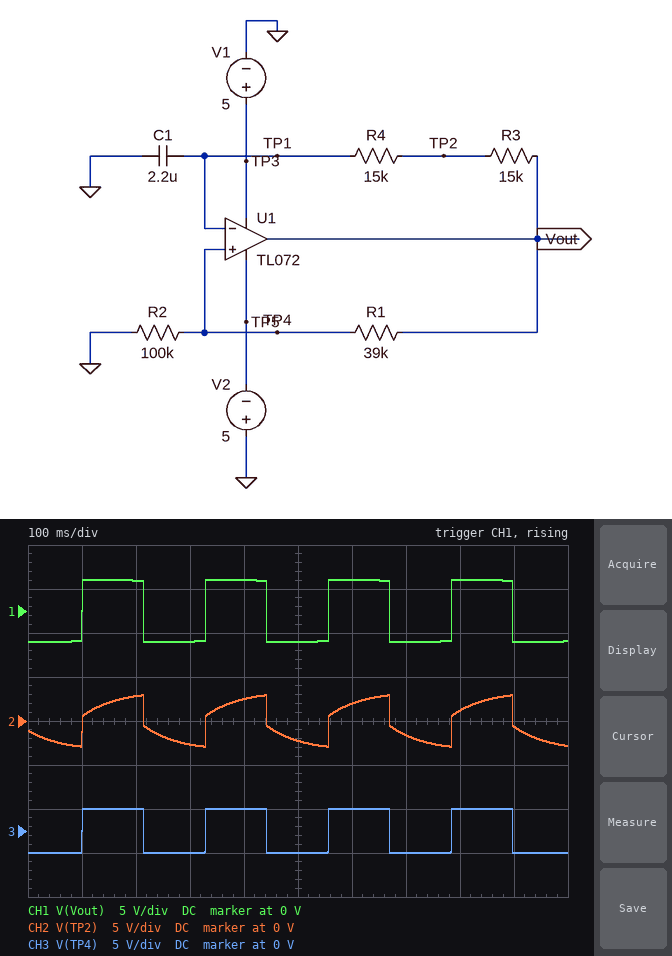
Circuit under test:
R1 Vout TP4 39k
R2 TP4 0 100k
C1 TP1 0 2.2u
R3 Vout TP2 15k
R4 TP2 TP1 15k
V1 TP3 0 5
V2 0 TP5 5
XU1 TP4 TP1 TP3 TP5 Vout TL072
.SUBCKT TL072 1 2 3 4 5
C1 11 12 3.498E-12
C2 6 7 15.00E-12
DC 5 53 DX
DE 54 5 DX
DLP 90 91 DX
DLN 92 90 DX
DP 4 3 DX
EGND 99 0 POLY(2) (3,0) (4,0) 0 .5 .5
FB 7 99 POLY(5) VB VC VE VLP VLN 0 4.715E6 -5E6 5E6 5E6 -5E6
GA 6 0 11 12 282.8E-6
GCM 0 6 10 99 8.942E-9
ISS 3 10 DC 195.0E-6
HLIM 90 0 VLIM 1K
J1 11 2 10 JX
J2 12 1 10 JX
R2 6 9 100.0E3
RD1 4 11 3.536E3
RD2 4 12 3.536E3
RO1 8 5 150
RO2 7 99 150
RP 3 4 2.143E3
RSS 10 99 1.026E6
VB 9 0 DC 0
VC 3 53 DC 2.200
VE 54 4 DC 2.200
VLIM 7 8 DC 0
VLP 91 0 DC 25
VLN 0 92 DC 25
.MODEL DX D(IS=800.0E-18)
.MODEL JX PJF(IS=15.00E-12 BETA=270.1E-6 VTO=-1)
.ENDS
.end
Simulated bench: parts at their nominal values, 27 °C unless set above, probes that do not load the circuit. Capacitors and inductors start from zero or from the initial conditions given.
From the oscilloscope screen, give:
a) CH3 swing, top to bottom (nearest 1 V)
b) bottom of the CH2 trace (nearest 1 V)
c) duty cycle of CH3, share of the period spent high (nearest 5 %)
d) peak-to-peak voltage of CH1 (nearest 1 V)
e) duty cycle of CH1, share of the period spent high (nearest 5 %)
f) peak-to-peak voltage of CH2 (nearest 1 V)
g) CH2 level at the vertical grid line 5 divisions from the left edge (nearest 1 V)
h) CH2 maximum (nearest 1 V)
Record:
5 V
-3 V
50 %
7 V
50 %
6 V
-2 V
3 V
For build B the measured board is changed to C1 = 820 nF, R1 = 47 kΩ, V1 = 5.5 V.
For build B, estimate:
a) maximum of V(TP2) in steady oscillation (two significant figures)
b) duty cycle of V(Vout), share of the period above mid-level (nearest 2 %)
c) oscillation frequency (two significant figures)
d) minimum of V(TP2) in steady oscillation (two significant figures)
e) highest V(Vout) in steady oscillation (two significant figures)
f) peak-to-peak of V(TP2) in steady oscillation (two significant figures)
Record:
3.3 V
48 %
13 Hz
-2.8 V
4.0 V
6.1 V
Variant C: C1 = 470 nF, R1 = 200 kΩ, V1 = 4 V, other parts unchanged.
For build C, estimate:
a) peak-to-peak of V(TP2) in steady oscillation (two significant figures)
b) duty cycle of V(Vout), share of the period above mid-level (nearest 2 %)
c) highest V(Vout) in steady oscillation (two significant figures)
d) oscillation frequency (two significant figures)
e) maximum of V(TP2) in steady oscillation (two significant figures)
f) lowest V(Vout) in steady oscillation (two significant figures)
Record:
3.8 V
56 %
2.5 V
53 Hz
1.6 V
-3.5 V
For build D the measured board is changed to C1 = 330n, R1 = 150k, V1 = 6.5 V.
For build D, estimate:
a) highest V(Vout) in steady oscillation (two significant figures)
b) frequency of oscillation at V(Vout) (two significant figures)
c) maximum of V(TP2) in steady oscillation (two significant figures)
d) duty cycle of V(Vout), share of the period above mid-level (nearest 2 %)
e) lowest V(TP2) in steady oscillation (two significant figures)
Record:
5.0 V
61 Hz
3.4 V
44 %
-2.4 V
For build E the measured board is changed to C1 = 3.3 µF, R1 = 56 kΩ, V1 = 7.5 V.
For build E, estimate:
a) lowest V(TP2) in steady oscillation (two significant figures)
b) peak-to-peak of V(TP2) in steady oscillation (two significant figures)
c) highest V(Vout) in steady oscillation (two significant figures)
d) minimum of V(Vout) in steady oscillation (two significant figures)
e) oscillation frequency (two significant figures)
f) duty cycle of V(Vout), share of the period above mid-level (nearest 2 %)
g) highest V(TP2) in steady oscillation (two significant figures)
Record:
-2.8 V
7.6 V
6.0 V
-3.5 V
3.4 Hz
44 %
4.8 V
